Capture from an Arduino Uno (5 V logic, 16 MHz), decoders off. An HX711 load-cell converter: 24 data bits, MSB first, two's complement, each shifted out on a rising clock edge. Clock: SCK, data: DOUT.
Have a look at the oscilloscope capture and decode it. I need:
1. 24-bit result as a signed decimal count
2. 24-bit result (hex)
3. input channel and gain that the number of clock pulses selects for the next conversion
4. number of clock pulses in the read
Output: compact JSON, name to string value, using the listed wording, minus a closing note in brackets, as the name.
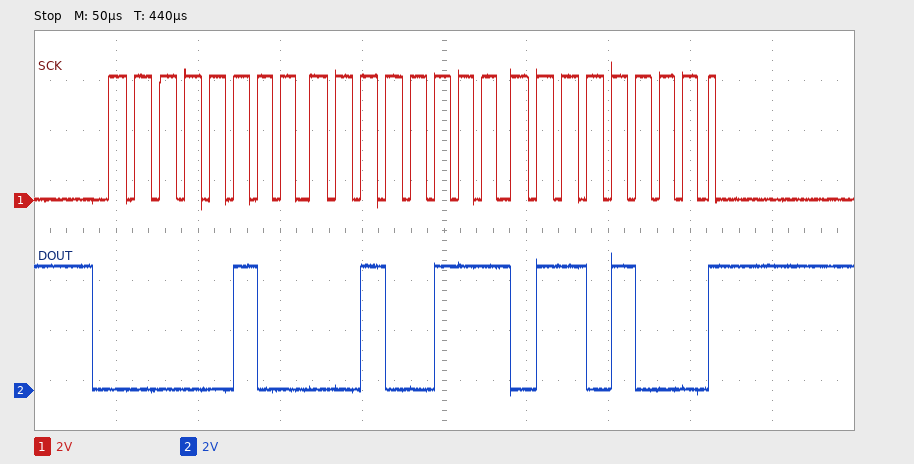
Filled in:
{"24-bit result as a signed decimal count": "272232", "24-bit result": "0x042768", "input channel and gain that the number of clock pulses selects for the next conversion": "channel A, gain 128", "number of clock pulses in the read": "25"}
